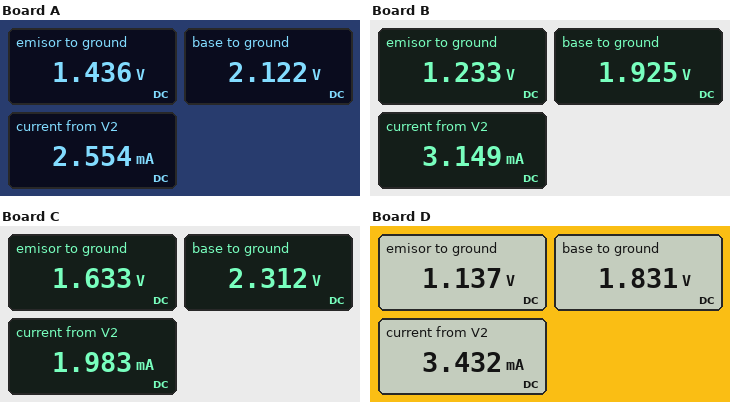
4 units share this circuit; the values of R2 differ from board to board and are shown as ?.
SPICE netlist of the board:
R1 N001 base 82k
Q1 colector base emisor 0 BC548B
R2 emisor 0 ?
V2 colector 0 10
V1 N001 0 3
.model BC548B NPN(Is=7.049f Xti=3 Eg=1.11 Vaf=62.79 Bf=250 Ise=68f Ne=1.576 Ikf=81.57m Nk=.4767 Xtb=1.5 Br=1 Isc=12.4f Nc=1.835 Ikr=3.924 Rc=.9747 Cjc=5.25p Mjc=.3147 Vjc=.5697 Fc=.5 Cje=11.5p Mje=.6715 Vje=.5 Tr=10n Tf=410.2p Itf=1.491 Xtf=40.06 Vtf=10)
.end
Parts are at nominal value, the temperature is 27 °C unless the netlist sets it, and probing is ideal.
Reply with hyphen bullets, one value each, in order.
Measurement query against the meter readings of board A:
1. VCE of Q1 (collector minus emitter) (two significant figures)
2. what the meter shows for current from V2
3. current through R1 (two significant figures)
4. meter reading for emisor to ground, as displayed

- 8.6 V
- 2.554 mA
- 11 µA
- 1.436 V
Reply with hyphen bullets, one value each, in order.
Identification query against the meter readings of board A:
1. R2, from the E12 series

- 560 Ω
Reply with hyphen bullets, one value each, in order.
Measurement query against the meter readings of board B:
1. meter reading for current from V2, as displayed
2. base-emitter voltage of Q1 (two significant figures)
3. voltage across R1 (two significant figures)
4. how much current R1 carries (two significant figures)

- 3.149 mA
- 690 mV
- 1.1 V
- 13 µA
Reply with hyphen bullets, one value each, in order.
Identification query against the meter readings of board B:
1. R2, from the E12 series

- 390 Ω
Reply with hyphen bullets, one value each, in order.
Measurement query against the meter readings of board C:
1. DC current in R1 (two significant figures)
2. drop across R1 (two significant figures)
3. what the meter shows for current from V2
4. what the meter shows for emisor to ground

- 8.4 µA
- 690 mV
- 1.983 mA
- 1.633 V
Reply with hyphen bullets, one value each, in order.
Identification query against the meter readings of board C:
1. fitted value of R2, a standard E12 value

- 820 Ω
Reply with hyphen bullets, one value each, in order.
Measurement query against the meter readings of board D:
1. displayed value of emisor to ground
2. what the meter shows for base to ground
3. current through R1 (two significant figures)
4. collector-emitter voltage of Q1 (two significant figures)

- 1.137 V
- 1.831 V
- 14 µA
- 8.9 V
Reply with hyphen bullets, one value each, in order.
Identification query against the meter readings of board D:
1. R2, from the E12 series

- 330 Ω
